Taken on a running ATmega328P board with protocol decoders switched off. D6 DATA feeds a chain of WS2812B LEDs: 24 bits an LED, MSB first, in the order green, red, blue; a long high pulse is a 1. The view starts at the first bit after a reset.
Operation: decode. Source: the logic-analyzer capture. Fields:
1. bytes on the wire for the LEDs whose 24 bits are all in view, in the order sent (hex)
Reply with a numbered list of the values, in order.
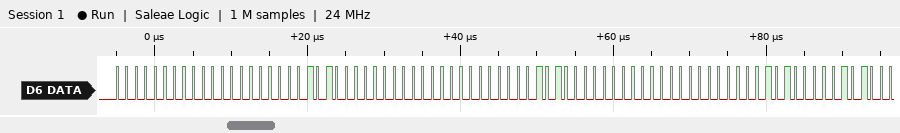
1. 00 00 0A 00 00 0A 00 00 0A
